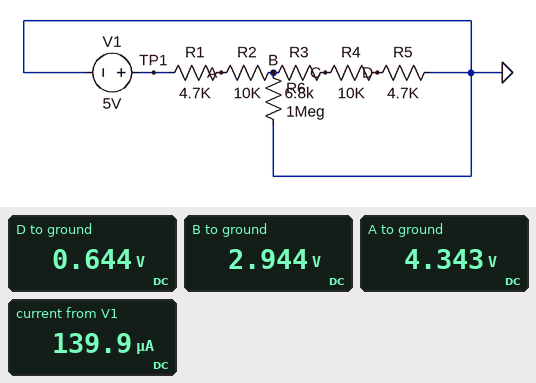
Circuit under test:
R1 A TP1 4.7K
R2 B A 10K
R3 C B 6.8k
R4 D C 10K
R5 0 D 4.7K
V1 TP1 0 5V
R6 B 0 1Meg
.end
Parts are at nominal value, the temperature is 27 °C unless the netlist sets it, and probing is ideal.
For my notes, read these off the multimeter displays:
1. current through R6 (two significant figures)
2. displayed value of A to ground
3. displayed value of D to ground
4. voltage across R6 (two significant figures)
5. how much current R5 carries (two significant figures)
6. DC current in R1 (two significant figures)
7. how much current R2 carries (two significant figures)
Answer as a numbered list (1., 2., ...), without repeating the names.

1. 2.9 µA
2. 4.343 V
3. 0.644 V
4. 2.9 V
5. 140 µA
6. 140 µA
7. 140 µA
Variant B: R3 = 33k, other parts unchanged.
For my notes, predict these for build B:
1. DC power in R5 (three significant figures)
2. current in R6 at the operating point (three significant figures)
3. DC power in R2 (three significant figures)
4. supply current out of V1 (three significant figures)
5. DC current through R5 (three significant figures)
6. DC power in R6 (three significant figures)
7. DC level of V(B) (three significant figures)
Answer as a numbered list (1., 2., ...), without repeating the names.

1. 29.5 µW
2. 3.78 µA
3. 68.9 µW
4. 83.0 µA
5. 79.2 µA
6. 14.3 µW
7. 3.78 V
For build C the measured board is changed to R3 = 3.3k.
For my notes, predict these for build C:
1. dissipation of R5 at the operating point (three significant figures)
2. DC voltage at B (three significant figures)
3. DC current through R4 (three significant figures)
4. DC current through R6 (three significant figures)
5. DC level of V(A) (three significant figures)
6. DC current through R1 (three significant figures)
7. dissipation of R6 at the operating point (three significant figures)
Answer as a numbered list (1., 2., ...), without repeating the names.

1. 108 µW
2. 2.73 V
3. 152 µA
4. 2.73 µA
5. 4.27 V
6. 154 µA
7. 7.45 µW
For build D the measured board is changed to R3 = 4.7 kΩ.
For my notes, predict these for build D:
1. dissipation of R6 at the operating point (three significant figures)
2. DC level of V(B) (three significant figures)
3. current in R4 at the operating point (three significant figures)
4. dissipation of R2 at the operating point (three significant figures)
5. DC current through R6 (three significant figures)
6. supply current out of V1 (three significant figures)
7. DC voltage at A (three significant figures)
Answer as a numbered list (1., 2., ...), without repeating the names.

1. 7.96 µW
2. 2.82 V
3. 145 µA
4. 220 µW
5. 2.82 µA
6. 148 µA
7. 4.30 V
